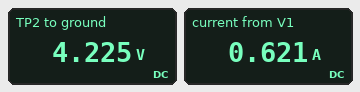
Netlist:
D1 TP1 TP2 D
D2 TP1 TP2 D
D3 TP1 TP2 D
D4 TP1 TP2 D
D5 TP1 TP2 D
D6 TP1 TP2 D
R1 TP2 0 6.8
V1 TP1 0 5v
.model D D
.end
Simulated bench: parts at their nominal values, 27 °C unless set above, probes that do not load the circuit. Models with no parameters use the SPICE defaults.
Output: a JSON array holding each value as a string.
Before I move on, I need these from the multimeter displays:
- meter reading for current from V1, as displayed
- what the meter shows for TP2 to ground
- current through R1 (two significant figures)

["0.621 A", "4.225 V", "620 mA"]
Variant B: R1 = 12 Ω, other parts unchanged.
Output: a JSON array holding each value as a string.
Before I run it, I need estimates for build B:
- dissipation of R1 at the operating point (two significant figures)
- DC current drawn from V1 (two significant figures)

["1.5 W", "350 mA"]
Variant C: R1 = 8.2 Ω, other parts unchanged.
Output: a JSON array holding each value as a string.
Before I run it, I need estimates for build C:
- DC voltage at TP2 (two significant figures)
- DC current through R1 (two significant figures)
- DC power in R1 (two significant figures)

["4.2 V", "520 mA", "2.2 W"]
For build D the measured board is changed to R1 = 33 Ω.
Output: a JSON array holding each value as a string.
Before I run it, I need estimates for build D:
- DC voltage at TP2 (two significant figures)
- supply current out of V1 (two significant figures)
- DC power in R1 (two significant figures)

["4.3 V", "130 mA", "550 mW"]
